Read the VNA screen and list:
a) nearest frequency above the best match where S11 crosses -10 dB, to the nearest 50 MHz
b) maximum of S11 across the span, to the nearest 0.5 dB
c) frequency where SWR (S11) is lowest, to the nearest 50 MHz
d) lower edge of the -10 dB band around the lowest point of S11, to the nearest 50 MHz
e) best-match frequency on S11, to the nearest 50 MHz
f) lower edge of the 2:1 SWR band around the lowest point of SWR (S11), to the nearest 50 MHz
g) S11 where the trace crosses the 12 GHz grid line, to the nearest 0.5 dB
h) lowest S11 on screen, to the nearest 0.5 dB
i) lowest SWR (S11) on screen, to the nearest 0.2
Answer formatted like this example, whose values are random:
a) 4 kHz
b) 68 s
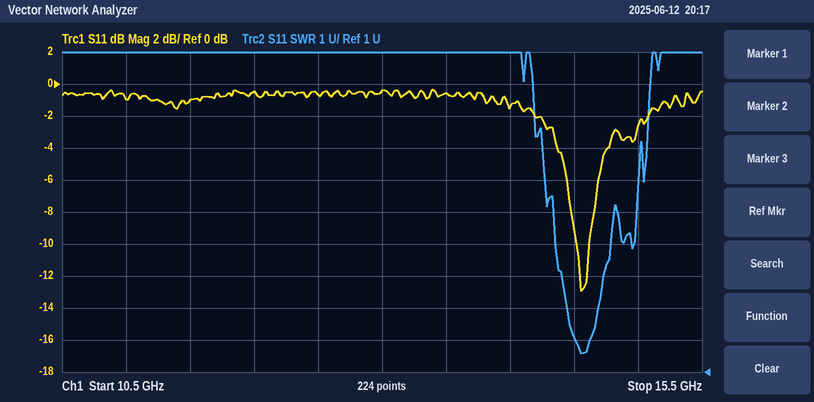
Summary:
a) 14.60 GHz
b) -0.5 dB
c) 14.55 GHz
d) 14.50 GHz
e) 14.55 GHz
f) 14.50 GHz
g) -0.5 dB
h) -13.0 dB
i) 1.6
